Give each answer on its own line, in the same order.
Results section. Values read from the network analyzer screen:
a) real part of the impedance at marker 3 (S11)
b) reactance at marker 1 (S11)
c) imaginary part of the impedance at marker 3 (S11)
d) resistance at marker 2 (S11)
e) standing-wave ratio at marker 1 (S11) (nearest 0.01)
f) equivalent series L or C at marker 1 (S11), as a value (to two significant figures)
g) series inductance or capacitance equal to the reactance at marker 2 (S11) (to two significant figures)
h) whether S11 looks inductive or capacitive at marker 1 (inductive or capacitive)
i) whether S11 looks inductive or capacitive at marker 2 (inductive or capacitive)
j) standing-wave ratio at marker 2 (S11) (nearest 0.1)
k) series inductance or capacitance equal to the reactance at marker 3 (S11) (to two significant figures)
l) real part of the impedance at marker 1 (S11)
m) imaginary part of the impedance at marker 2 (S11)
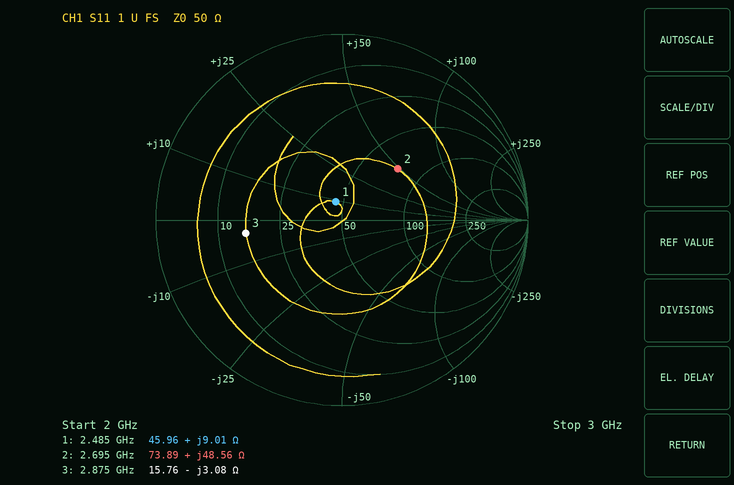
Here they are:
15.76 Ω
+9.01 Ω
-3.08 Ω
73.89 Ω
1.23
580 pH
2.9 nH
inductive
inductive
2.4
18 pF
45.96 Ω
+48.56 Ω
